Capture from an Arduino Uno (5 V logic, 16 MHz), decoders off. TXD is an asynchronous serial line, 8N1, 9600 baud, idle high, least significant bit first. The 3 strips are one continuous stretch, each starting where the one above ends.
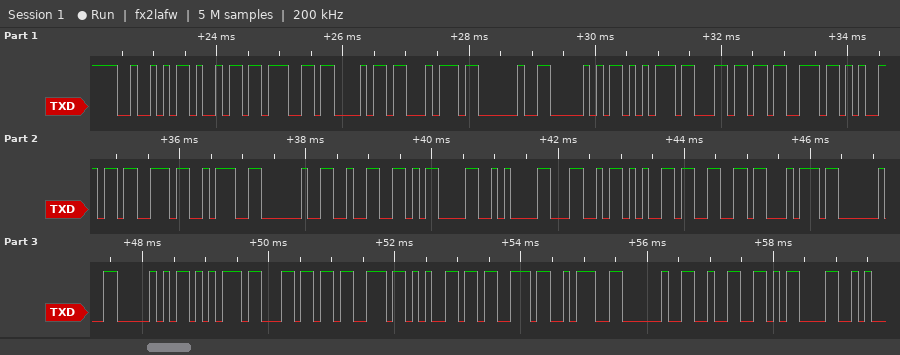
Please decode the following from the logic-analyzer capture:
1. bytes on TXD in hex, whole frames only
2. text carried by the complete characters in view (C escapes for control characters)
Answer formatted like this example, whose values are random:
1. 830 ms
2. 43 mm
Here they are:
1. 0x52 0x69 0x67 0x68 0x74 0x20 0x50 0x75 0x6C 0x73 0x65 0x73 0x3A 0x20 0x32 0x0D 0x0A 0x4C 0x65 0x66 0x74 0x20 0x50 0x75 0x6C 0x73 0x65 0x73 0x3A 0x20 0x32 0x0D
2. "Right Pulses: 2\r\nLeft Pulses: 2\r"
